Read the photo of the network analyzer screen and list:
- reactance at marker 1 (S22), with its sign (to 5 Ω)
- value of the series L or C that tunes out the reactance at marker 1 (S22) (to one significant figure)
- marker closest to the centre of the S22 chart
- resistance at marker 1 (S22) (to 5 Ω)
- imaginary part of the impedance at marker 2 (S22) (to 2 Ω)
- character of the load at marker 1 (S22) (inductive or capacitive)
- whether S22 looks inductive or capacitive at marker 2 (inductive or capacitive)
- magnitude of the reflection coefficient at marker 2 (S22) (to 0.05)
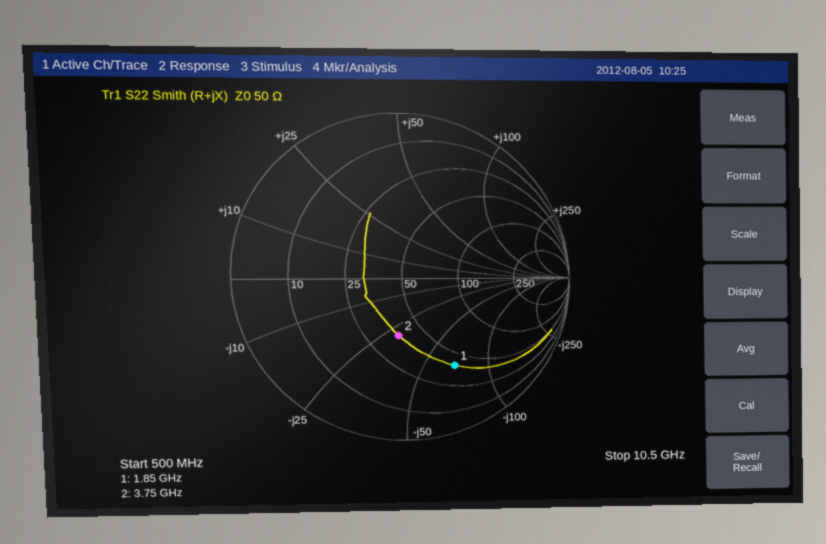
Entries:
-70 Ω
6 nH
marker 2
40 Ω
-30 Ω
capacitive
capacitive
0.35
